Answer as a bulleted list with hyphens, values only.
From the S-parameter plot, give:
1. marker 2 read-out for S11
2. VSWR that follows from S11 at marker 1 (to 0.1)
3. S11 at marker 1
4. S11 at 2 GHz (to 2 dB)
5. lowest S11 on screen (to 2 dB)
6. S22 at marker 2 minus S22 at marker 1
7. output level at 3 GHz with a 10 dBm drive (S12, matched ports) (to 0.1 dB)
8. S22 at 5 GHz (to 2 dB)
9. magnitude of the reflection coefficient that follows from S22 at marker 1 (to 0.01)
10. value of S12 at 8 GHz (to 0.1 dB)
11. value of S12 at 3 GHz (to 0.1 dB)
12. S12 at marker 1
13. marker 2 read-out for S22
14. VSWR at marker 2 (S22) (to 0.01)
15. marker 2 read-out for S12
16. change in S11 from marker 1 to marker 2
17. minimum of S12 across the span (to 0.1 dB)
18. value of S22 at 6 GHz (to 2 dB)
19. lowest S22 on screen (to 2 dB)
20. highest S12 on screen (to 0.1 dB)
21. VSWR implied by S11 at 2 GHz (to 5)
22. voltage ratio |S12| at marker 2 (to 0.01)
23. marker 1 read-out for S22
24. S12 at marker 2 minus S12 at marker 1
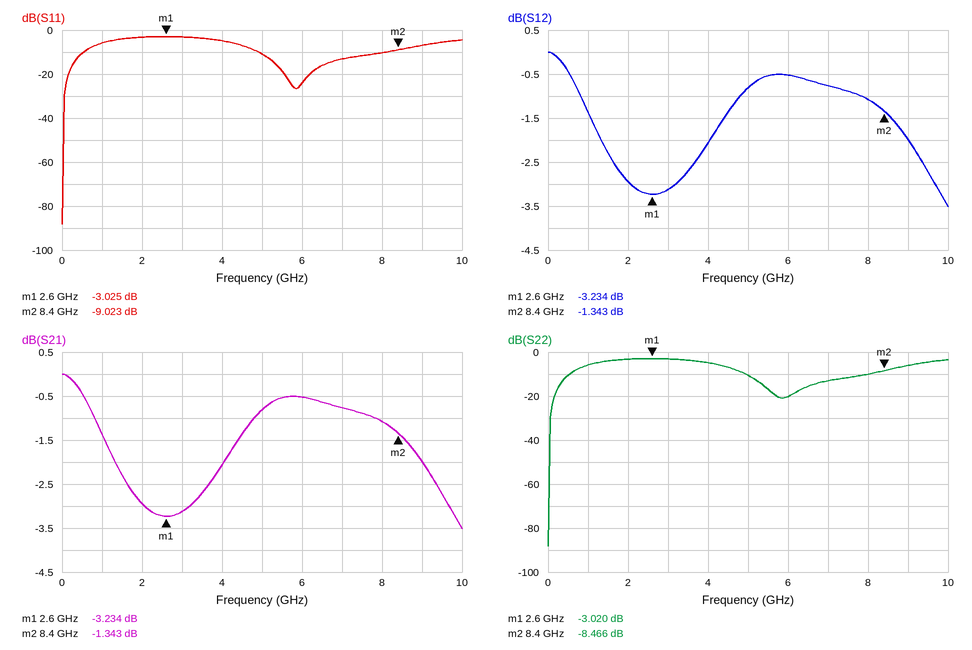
- -9.023 dB
- 5.8
- -3.025 dB
- -4 dB
- -88 dB
- -5.446 dB
- 6.9 dBm
- -10 dB
- 0.71
- -1.1 dB
- -3.1 dB
- -3.234 dB
- -8.466 dB
- 2.21
- -1.343 dB
- -5.998 dB
- -3.5 dB
- -20 dB
- -88 dB
- 0.0 dB
- 5
- 0.86
- -3.020 dB
- 1.891 dB
